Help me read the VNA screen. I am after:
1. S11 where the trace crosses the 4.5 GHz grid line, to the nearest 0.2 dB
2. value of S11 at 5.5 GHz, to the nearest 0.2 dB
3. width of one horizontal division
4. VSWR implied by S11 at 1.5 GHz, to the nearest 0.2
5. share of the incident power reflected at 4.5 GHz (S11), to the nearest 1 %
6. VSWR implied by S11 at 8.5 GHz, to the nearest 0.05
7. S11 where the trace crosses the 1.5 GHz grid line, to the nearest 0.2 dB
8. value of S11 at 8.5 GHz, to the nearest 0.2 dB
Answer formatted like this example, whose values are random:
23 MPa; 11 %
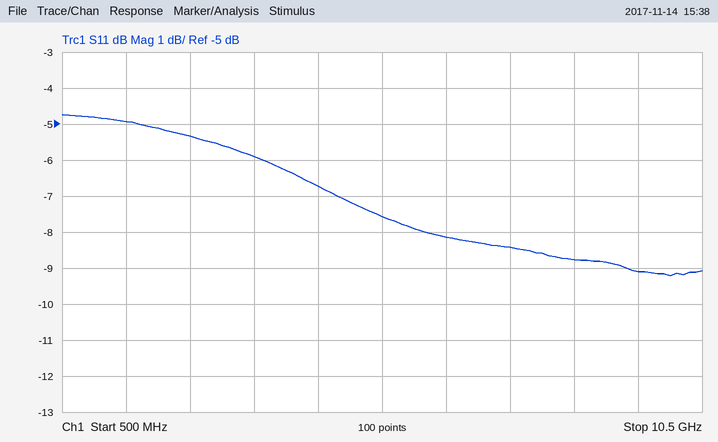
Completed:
-6.8 dB; -7.6 dB; 1 GHz; 3.6; 21 %; 2.15; -5.0 dB; -8.8 dB
